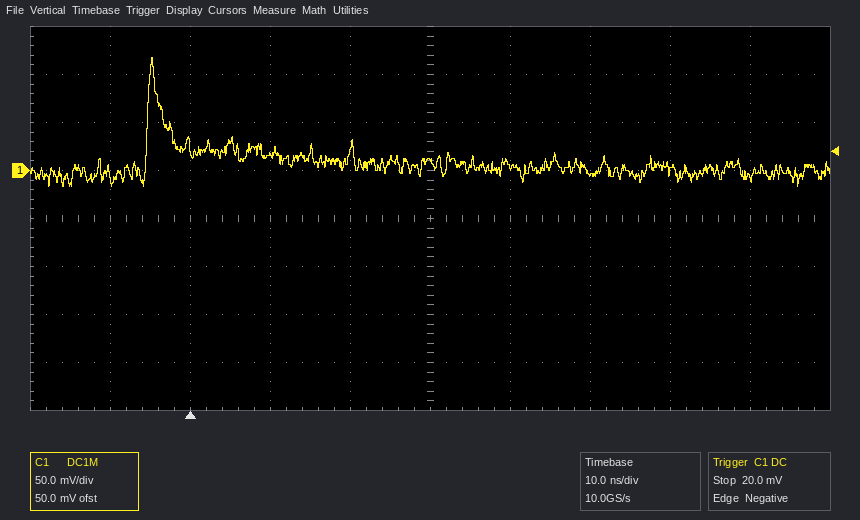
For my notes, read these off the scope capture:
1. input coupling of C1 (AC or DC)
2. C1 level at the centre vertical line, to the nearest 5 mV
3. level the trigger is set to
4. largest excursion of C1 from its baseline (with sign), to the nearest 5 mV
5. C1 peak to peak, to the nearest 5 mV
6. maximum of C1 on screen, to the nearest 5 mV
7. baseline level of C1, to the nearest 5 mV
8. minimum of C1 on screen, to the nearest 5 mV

DC
10 mV
20.0 mV
+115 mV
135 mV
120 mV
5 mV
-15 mV
